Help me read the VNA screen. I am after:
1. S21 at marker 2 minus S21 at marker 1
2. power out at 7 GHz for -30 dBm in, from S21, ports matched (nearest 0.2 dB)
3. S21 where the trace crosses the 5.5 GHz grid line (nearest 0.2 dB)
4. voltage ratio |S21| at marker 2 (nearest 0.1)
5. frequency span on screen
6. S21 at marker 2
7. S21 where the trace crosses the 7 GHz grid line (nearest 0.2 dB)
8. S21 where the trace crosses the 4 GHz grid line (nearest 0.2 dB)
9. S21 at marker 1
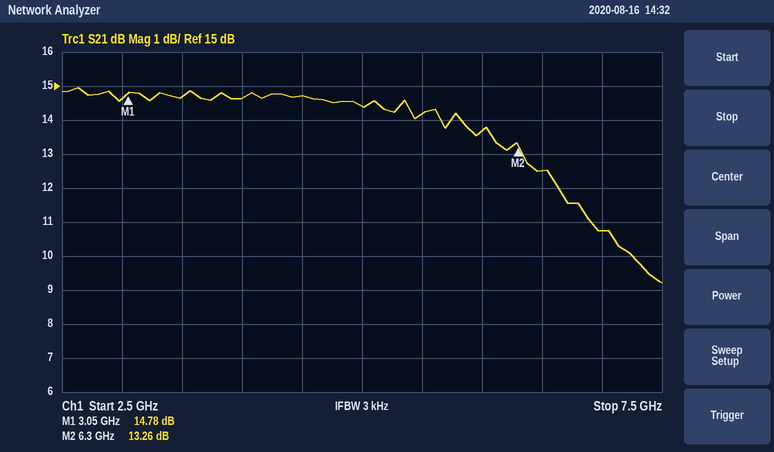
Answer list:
-1.52 dB
-19.2 dBm
14.2 dB
4.6
5 GHz
13.26 dB
10.8 dB
14.6 dB
14.78 dB
